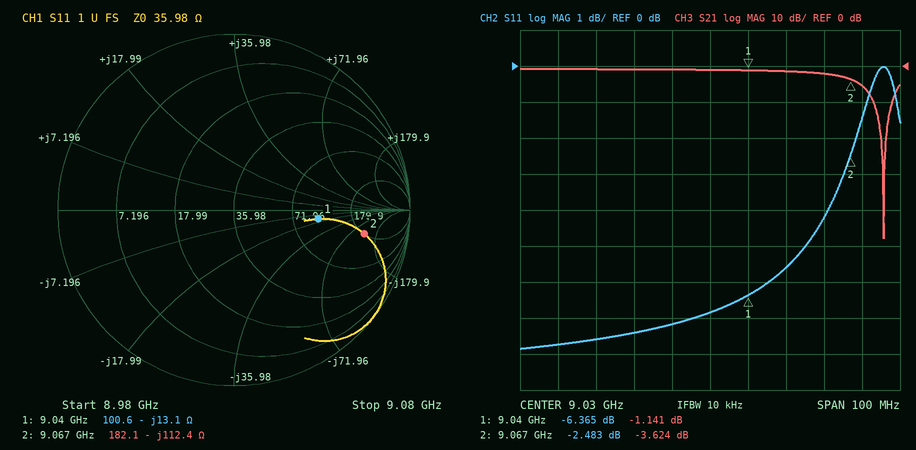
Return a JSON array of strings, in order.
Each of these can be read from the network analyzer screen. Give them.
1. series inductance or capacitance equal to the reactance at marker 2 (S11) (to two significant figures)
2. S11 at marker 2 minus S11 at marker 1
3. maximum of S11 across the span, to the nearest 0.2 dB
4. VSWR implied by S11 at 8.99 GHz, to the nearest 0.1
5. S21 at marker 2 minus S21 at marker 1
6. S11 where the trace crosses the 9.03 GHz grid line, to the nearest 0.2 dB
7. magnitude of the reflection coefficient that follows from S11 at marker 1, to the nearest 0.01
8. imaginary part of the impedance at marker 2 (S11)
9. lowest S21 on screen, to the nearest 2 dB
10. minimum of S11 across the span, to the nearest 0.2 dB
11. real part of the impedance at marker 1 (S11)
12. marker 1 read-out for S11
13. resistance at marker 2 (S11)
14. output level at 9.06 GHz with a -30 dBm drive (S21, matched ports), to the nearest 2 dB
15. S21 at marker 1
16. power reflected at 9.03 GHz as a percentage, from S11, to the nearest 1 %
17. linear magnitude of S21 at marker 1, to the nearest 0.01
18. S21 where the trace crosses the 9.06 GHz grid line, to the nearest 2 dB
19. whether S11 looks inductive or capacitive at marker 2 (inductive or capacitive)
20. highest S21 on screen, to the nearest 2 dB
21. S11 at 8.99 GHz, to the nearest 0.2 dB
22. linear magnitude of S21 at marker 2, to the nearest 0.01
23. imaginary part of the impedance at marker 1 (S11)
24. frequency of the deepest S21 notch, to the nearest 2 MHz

["160 fF", "3.882 dB", "0.0 dB", "2.4", "-2.483 dB", "-6.8 dB", "0.48", "-112.4 Ω", "-48 dB", "-7.8 dB", "100.6 Ω", "-6.365 dB", "182.1 Ω", "-32 dBm", "-1.141 dB", "21 %", "0.88", "-2 dB", "capacitive", "0 dB", "-7.8 dB", "0.66", "-13.1 Ω", "9.076 GHz"]
